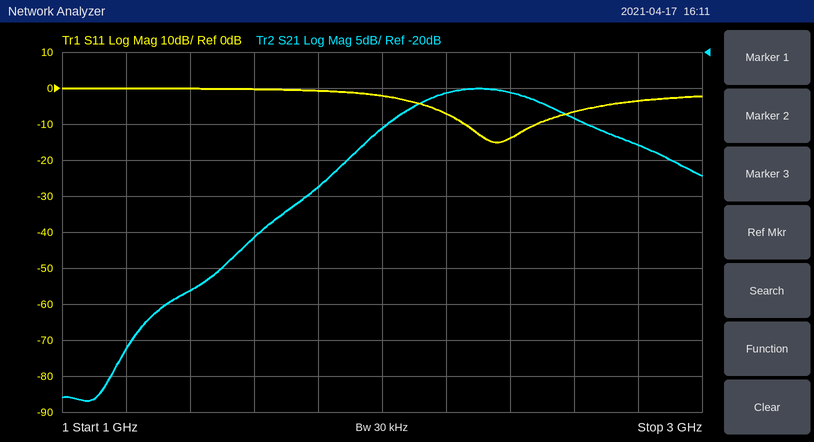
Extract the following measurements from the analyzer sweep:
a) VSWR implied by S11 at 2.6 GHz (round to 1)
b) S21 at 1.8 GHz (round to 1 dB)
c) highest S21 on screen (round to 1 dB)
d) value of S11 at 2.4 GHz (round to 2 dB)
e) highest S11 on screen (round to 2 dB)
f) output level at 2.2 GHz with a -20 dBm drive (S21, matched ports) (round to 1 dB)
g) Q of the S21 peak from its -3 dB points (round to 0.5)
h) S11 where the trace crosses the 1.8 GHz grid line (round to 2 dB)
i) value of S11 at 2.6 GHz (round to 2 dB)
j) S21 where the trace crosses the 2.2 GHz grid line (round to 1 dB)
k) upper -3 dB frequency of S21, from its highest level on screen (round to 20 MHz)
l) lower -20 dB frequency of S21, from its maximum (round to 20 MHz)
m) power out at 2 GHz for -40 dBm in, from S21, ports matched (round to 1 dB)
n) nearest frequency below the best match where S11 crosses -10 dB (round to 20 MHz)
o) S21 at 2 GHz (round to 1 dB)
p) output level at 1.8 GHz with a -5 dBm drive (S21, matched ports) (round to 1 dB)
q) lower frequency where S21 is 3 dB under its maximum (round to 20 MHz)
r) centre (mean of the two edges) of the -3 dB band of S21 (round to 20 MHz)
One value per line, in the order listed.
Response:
3
-39 dB
-25 dB
-14 dB
0 dB
-46 dBm
5.0
0 dB
-6 dB
-26 dB
2.54 GHz
1.62 GHz
-71 dBm
2.26 GHz
-31 dB
-44 dBm
2.08 GHz
2.32 GHz
